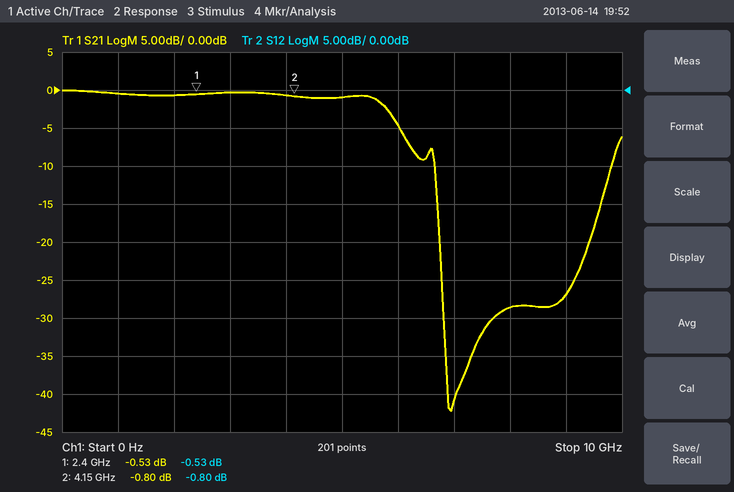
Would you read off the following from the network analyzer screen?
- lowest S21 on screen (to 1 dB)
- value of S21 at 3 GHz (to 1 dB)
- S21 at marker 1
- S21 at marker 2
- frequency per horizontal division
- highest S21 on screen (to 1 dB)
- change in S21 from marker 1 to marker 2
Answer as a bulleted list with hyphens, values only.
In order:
- -42 dB
- 0 dB
- -0.53 dB
- -0.80 dB
- 1 GHz
- 0 dB
- -0.27 dB
